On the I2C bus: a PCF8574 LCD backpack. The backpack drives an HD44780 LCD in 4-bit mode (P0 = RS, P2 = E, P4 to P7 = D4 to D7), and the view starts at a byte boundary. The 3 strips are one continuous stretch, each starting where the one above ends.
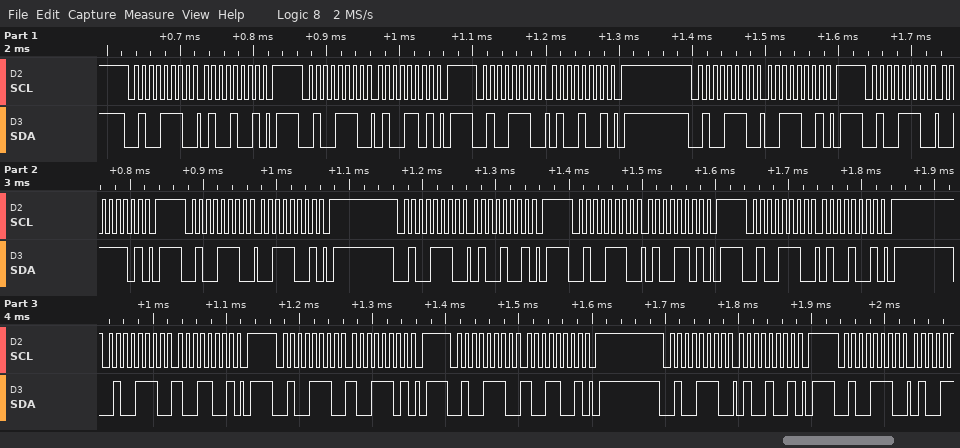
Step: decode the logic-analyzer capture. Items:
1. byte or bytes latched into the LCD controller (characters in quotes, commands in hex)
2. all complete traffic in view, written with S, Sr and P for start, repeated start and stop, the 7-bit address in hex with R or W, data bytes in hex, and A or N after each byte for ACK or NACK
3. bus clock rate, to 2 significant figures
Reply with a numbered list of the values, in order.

1. 'C' 'I'
2. S 27W A 49 A P S 27W A 4D A P S 27W A 49 A P S 27W A 39 A P S 27W A 3D A P S 27W A 39 A P S 27W A 49 A P S 27W A 4D A P S 27W A 49 A P S 27W A 99 A P S 27W A 9D A P S 27W A 99 A P S 27W A 49 A P S 27W A
3. 100 kHz
